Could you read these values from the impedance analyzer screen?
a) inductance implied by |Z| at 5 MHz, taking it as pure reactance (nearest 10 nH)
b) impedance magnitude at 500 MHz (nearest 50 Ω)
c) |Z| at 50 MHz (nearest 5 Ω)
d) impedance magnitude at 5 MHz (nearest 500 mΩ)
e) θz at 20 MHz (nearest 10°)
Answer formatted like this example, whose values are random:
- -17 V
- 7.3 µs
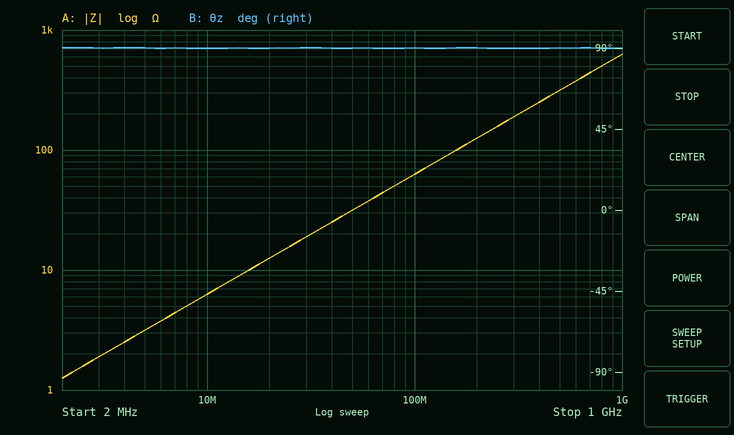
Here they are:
- 100 nH
- 300 Ω
- 30 Ω
- 3.0 Ω
- 90°
